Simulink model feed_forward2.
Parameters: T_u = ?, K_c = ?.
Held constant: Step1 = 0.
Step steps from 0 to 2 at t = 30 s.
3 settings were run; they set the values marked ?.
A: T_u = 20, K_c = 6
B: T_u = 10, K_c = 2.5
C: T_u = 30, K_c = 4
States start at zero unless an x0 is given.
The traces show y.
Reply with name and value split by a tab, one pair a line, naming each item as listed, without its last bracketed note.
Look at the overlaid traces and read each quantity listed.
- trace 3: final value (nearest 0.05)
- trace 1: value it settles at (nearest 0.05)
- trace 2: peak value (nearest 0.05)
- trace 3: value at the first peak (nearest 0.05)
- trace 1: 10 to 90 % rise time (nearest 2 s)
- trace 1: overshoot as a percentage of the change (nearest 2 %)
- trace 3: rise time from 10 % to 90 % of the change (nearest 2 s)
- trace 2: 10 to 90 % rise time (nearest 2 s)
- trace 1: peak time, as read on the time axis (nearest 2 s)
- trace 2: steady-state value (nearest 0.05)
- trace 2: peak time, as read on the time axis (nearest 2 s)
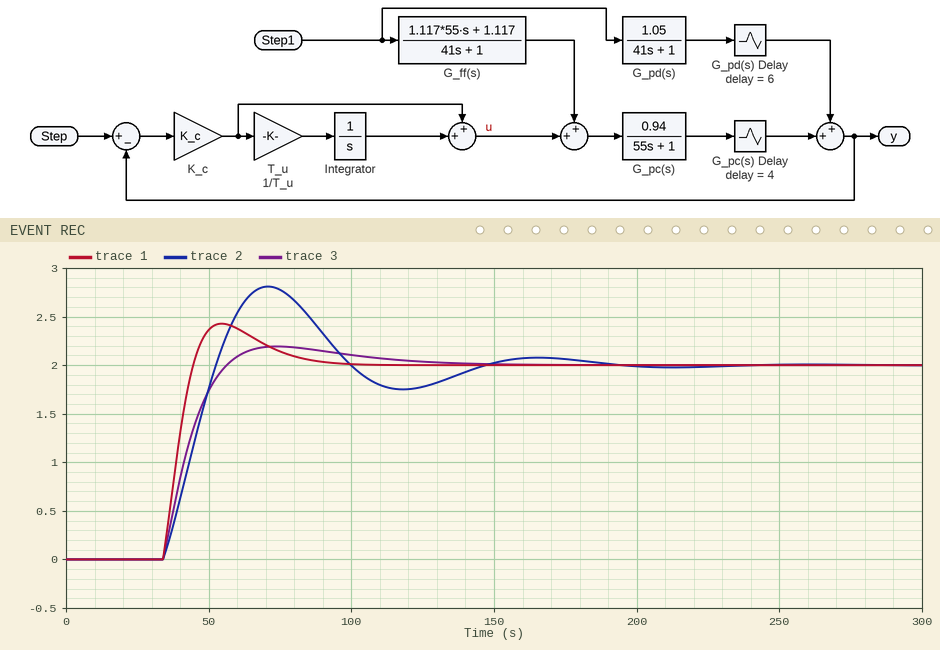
trace 3: final value	2.00
trace 1: value it settles at	2.00
trace 2: peak value	2.80
trace 3: value at the first peak	2.20
trace 1: 10 to 90 % rise time	8 s
trace 1: overshoot as a percentage of the change	22 %
trace 3: rise time from 10 % to 90 % of the change	16 s
trace 2: 10 to 90 % rise time	14 s
trace 1: peak time, as read on the time axis	54 s
trace 2: steady-state value	2.00
trace 2: peak time, as read on the time axis	70 s
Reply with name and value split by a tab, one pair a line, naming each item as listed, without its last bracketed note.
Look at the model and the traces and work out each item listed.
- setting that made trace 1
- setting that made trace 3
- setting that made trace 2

setting that made trace 1	A
setting that made trace 3	C
setting that made trace 2	B
